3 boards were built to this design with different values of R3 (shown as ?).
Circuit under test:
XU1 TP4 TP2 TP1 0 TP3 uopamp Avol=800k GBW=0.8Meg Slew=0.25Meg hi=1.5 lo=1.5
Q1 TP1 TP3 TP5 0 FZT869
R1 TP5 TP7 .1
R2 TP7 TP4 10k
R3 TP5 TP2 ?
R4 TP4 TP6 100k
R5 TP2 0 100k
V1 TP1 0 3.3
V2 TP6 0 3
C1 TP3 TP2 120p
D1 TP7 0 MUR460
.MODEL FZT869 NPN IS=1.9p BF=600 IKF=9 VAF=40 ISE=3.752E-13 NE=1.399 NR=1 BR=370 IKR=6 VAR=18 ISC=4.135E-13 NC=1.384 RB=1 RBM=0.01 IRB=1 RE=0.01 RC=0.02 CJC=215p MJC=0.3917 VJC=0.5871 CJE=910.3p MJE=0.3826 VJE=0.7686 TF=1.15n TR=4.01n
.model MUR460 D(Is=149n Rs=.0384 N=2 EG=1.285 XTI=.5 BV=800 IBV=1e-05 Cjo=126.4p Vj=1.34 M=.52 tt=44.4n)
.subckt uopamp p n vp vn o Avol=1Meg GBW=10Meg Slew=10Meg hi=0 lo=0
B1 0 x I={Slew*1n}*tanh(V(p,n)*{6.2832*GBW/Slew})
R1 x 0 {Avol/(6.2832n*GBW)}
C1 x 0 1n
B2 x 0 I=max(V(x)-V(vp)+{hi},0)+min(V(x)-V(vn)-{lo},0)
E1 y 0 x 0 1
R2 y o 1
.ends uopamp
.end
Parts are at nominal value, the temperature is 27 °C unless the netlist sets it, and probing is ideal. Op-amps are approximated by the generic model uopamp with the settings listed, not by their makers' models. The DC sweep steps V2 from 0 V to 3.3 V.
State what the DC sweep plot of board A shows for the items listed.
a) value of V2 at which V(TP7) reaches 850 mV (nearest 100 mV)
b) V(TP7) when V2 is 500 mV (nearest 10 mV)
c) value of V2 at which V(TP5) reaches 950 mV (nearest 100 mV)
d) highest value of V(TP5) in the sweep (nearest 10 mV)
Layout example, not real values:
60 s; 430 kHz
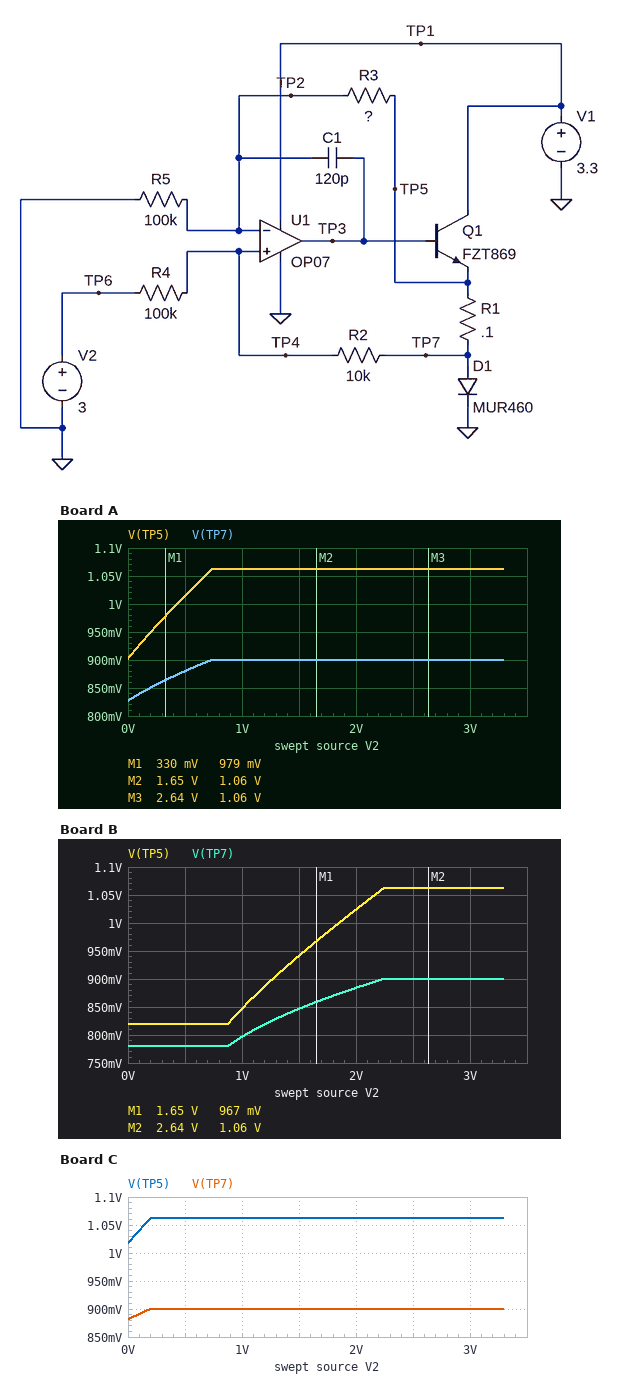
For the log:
200 mV; 880 mV; 200 mV; 1.06 V
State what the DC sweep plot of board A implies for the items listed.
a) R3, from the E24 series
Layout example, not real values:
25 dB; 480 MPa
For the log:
20 kΩ
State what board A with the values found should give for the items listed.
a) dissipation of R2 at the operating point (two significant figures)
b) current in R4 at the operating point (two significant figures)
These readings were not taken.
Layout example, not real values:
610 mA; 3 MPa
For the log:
3.6 µW; 19 µA
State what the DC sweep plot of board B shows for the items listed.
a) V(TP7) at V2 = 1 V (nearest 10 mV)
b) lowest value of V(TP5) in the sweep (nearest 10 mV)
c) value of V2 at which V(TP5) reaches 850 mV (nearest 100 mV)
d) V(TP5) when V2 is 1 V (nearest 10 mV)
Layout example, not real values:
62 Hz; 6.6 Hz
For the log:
800 mV; 820 mV; 1.0 V; 850 mV
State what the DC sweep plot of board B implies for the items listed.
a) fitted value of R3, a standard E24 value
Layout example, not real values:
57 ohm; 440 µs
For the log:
3.9 kΩ
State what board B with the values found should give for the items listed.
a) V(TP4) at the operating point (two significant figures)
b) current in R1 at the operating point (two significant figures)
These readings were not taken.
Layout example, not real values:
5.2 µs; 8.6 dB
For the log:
1.1 V; 1.6 A
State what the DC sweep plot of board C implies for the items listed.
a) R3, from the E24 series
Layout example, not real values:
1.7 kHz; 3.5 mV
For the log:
27 kΩ
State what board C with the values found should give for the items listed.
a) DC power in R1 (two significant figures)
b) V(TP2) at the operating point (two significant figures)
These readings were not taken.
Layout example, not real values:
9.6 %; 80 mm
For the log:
260 mW; 840 mV
